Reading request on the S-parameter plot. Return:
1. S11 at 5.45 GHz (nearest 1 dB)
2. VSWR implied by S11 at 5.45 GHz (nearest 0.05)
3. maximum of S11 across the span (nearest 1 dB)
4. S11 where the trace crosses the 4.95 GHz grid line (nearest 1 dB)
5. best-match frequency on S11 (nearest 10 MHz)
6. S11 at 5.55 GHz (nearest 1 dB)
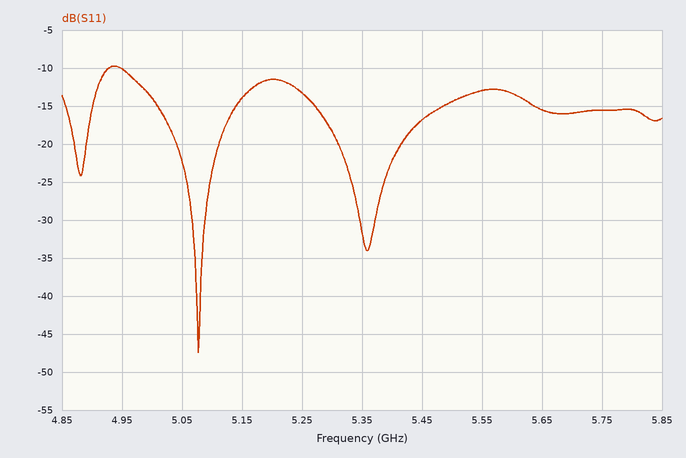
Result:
-17 dB
1.35
-10 dB
-10 dB
5.08 GHz
-13 dB
